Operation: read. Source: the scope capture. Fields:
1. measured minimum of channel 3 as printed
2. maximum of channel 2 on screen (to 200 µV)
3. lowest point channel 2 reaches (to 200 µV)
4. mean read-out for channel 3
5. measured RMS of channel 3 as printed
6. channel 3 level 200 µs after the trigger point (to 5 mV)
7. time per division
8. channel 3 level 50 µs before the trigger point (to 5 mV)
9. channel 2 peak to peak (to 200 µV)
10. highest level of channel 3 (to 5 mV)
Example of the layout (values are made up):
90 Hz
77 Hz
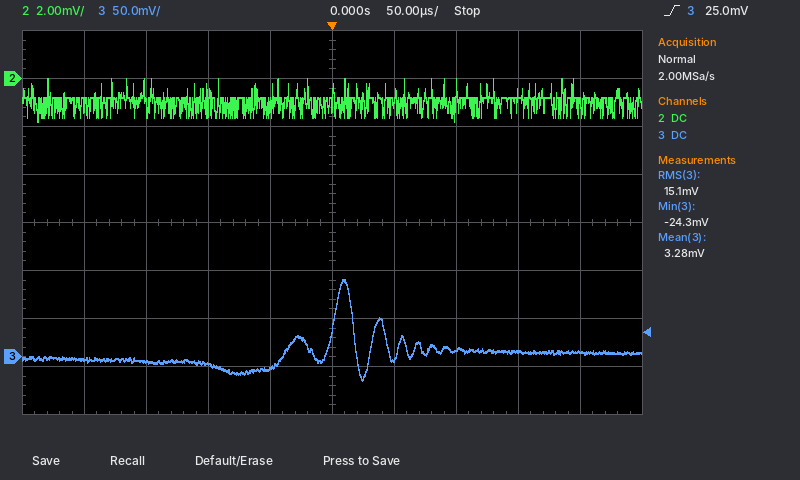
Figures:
-24.3 mV
0.0 mV
-1.8 mV
3.28 mV
15.1 mV
5 mV
50 µs
-10 mV
1.8 mV
80 mV
